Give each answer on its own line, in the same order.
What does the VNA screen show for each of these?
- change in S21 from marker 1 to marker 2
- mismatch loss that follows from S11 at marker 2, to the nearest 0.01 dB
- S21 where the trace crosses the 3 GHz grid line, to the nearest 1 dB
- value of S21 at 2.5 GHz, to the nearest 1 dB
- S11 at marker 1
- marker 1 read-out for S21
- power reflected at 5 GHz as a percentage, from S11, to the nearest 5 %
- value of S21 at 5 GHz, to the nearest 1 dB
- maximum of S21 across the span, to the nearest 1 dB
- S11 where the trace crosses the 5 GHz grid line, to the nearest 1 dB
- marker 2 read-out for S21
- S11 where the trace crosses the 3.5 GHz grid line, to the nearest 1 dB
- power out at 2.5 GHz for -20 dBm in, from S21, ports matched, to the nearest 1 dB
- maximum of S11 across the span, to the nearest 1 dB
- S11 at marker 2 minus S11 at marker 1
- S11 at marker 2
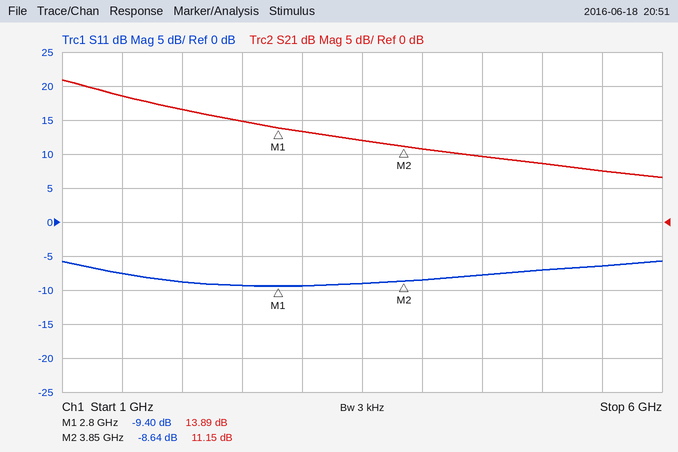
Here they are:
-2.74 dB
0.64 dB
13 dB
15 dB
-9.40 dB
13.89 dB
20 %
9 dB
21 dB
-7 dB
11.15 dB
-9 dB
-5 dBm
-6 dB
0.76 dB
-8.64 dB
